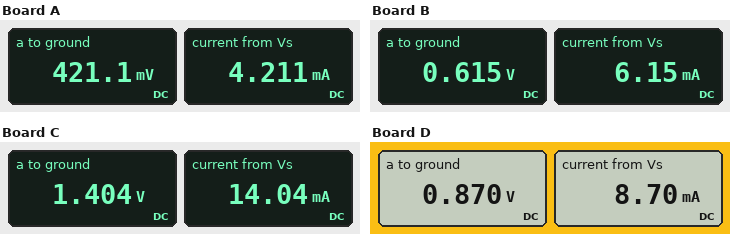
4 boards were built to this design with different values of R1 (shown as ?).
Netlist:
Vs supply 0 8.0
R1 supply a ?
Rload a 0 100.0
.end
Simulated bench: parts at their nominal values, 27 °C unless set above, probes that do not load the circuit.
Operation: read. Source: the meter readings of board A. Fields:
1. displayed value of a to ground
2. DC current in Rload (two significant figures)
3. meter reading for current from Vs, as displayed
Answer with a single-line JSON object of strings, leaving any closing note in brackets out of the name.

{"displayed value of a to ground": "421.1 mV", "DC current in Rload": "4.2 mA", "meter reading for current from Vs, as displayed": "4.211 mA"}
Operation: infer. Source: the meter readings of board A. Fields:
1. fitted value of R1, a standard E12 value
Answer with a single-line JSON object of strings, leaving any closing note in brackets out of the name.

{"fitted value of R1, a standard E12 value": "1.8 kΩ"}
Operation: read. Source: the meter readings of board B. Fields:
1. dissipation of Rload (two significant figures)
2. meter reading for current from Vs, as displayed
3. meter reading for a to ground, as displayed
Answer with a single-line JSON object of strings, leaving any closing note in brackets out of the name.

{"dissipation of Rload": "3.8 mW", "meter reading for current from Vs, as displayed": "6.15 mA", "meter reading for a to ground, as displayed": "0.615 V"}
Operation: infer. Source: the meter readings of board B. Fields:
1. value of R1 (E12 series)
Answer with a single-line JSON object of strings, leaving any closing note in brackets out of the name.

{"value of R1": "1.2 kΩ"}
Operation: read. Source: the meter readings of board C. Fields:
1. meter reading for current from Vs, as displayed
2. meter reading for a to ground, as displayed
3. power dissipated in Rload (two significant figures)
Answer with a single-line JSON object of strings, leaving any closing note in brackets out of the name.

{"meter reading for current from Vs, as displayed": "14.04 mA", "meter reading for a to ground, as displayed": "1.404 V", "power dissipated in Rload": "20 mW"}
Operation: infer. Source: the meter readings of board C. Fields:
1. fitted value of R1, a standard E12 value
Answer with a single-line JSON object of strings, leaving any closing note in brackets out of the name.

{"fitted value of R1, a standard E12 value": "470 Ω"}
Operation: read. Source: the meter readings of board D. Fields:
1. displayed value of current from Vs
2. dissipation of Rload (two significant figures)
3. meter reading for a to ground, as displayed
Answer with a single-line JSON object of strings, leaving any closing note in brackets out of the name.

{"displayed value of current from Vs": "8.70 mA", "dissipation of Rload": "7.6 mW", "meter reading for a to ground, as displayed": "0.870 V"}
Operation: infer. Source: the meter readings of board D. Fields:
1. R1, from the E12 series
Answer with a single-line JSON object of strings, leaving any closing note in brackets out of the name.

{"R1, from the E12 series": "820 Ω"}
